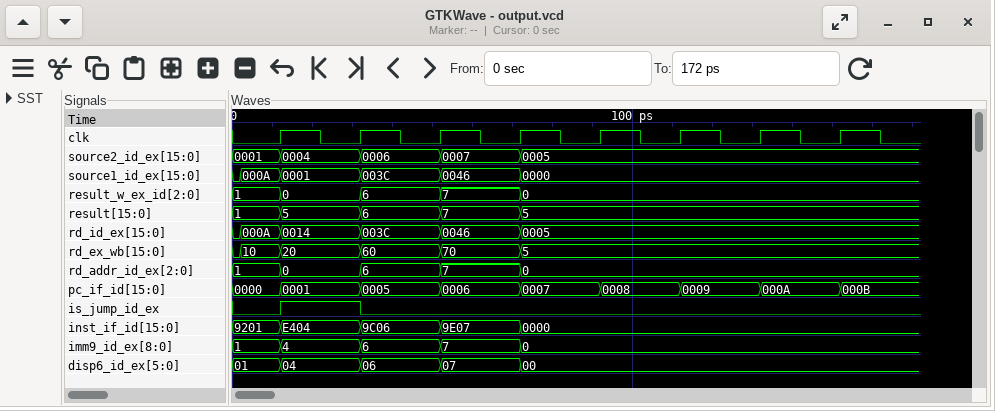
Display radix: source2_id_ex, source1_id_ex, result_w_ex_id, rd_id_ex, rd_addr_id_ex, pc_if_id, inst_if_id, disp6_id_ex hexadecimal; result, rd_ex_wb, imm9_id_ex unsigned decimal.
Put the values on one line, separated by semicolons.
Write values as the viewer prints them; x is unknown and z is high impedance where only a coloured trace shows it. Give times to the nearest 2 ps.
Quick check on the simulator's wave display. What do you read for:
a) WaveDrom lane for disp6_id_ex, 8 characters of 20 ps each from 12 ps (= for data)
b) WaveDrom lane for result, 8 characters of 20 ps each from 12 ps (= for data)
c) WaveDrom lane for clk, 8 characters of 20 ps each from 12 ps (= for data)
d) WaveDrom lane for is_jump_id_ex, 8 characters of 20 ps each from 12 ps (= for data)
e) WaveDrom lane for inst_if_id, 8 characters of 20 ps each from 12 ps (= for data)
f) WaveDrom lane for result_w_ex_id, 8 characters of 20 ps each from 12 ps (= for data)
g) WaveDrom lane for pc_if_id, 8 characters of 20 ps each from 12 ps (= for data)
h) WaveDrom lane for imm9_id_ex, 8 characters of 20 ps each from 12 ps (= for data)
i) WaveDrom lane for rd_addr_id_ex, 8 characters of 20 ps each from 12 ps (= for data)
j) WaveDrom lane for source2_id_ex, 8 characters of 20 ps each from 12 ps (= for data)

{name: 'disp6_id_ex', wave: '====....', data: '04 06 07 00'}; {name: 'result', wave: '====....', data: '5 6 7 5'}; {name: 'clk', wave: 'p.......'}; {name: 'is_jump_id_ex', wave: '10......'}; {name: 'inst_if_id', wave: '====....', data: 'E404 9C06 9E07 0000'}; {name: 'result_w_ex_id', wave: '====....', data: '0 6 7 0'}; {name: 'pc_if_id', wave: '========', data: '0001 0005 0006 0007 0008 0009 000A 000B'}; {name: 'imm9_id_ex', wave: '====....', data: '4 6 7 0'}; {name: 'rd_addr_id_ex', wave: '====....', data: '0 6 7 0'}; {name: 'source2_id_ex', wave: '====....', data: '0004 0006 0007 0005'}
